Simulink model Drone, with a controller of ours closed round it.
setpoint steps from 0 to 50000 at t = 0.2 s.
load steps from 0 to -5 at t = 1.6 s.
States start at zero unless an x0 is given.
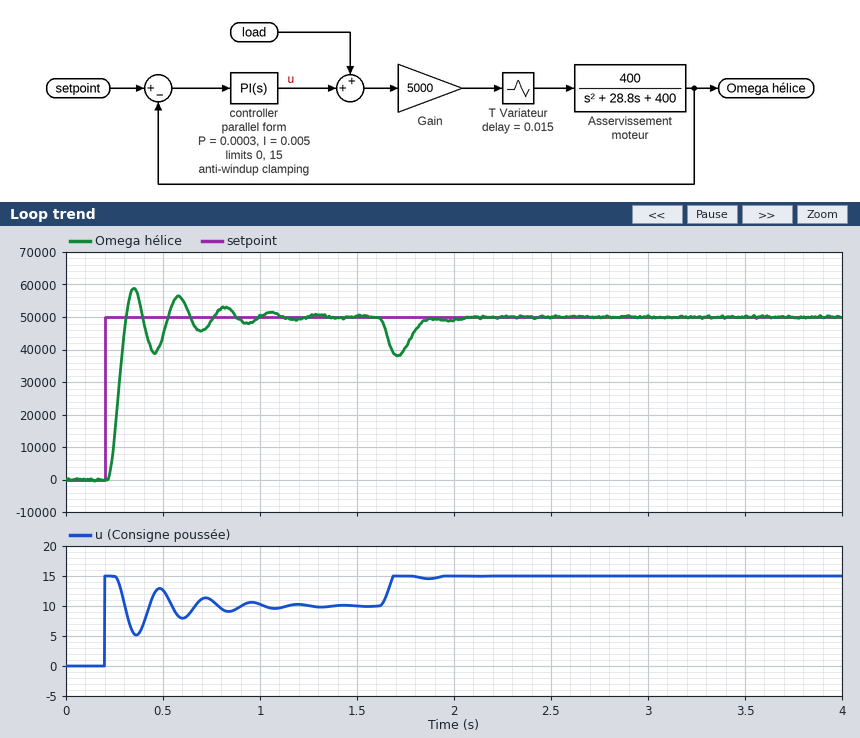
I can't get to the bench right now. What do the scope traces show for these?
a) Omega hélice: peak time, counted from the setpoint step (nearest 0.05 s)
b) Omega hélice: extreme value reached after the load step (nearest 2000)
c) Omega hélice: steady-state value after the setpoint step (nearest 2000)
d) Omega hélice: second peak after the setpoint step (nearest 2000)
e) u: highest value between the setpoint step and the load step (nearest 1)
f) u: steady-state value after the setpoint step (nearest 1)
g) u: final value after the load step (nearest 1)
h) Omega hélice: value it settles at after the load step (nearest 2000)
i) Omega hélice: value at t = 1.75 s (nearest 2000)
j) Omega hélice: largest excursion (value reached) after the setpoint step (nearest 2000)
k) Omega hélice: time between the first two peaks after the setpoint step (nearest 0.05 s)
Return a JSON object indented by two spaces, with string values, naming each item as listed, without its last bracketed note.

{
  "Omega hélice: peak time, counted from the setpoint step": "0.15 s",
  "Omega hélice: extreme value reached after the load step": "38000",
  "Omega hélice: steady-state value after the setpoint step": "50000",
  "Omega hélice: second peak after the setpoint step": "56000",
  "u: highest value between the setpoint step and the load step": "15",
  "u: steady-state value after the setpoint step": "10",
  "u: final value after the load step": "15",
  "Omega hélice: value it settles at after the load step": "50000",
  "Omega hélice: value at t = 1.75 s": "40000",
  "Omega hélice: largest excursion (value reached) after the setpoint step": "58000",
  "Omega hélice: time between the first two peaks after the setpoint step": "0.25 s"
}
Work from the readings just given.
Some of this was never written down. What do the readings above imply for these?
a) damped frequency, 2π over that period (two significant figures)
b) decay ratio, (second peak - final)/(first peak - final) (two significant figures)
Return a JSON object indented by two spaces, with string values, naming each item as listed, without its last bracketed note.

{
  "damped frequency, 2π over that period": "25 rad/s",
  "decay ratio, (second peak - final)/(first peak - final)": "0.75"
}
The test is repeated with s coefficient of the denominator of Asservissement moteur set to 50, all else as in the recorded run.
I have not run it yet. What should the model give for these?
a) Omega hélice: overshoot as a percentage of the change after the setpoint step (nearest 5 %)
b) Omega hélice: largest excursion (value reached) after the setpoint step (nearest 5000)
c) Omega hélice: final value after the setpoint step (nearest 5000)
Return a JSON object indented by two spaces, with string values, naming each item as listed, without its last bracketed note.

{
  "Omega hélice: overshoot as a percentage of the change after the setpoint step": "10 %",
  "Omega hélice: largest excursion (value reached) after the setpoint step": "55000",
  "Omega hélice: final value after the setpoint step": "50000"
}
